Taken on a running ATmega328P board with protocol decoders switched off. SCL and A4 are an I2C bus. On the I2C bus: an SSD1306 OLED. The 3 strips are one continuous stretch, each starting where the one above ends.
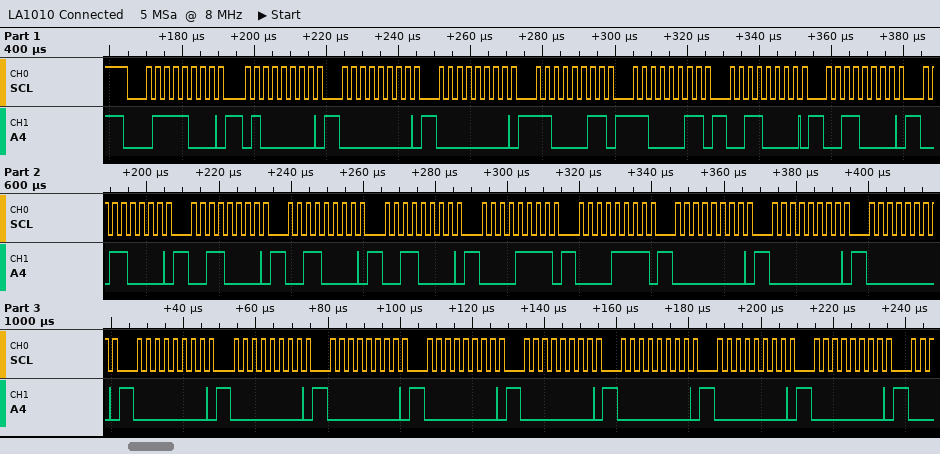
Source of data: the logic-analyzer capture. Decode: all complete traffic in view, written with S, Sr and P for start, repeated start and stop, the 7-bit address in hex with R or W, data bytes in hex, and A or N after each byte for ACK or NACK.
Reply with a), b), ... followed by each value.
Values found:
a) S 3CW A 40 A 00 A 00 A C3 A C3 A 30 A 30 A 30 A 30 A 30 A 30 A 0F A 0F A 00 A 00 A 00 A 00 A 00 A 00 A 00 A 00 A 00 A 00 A 00 A
